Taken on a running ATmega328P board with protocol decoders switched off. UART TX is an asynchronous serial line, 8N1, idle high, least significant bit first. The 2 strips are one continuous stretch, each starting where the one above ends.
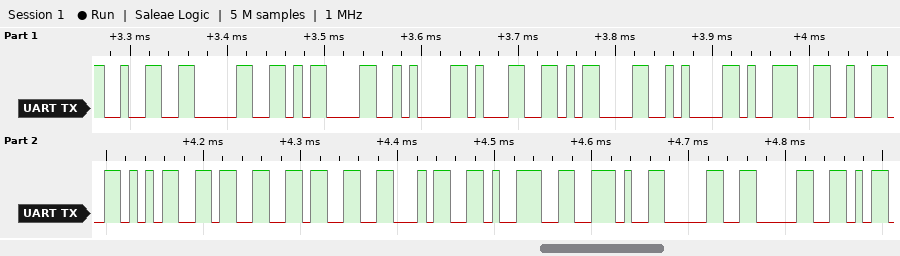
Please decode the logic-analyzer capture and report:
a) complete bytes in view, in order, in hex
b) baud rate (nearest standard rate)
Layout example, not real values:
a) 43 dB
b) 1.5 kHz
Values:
a) 32 30 0D 0A 31 0D 0A 39 32 35 33 33 34 39 2E 30 30
b) 115200 baud
